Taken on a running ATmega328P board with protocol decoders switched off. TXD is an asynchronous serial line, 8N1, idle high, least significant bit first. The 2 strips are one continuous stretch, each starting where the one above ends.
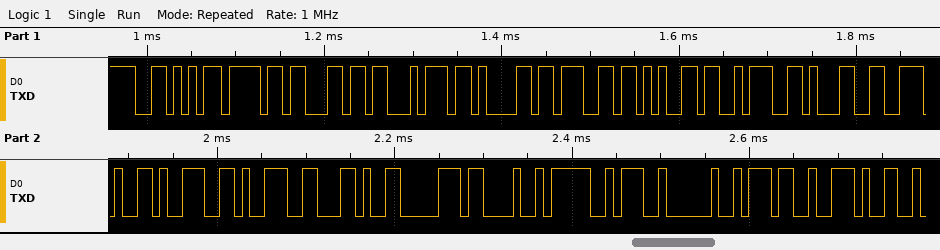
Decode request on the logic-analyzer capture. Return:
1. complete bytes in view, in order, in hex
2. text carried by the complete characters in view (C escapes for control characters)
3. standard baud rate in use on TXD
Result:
56 6F 6C 74 61 67 65 3A 31 2E 39 39 2C 70 48 3A 20 37 2E
"Voltage:1.99,pH: 7."
115200 baud
